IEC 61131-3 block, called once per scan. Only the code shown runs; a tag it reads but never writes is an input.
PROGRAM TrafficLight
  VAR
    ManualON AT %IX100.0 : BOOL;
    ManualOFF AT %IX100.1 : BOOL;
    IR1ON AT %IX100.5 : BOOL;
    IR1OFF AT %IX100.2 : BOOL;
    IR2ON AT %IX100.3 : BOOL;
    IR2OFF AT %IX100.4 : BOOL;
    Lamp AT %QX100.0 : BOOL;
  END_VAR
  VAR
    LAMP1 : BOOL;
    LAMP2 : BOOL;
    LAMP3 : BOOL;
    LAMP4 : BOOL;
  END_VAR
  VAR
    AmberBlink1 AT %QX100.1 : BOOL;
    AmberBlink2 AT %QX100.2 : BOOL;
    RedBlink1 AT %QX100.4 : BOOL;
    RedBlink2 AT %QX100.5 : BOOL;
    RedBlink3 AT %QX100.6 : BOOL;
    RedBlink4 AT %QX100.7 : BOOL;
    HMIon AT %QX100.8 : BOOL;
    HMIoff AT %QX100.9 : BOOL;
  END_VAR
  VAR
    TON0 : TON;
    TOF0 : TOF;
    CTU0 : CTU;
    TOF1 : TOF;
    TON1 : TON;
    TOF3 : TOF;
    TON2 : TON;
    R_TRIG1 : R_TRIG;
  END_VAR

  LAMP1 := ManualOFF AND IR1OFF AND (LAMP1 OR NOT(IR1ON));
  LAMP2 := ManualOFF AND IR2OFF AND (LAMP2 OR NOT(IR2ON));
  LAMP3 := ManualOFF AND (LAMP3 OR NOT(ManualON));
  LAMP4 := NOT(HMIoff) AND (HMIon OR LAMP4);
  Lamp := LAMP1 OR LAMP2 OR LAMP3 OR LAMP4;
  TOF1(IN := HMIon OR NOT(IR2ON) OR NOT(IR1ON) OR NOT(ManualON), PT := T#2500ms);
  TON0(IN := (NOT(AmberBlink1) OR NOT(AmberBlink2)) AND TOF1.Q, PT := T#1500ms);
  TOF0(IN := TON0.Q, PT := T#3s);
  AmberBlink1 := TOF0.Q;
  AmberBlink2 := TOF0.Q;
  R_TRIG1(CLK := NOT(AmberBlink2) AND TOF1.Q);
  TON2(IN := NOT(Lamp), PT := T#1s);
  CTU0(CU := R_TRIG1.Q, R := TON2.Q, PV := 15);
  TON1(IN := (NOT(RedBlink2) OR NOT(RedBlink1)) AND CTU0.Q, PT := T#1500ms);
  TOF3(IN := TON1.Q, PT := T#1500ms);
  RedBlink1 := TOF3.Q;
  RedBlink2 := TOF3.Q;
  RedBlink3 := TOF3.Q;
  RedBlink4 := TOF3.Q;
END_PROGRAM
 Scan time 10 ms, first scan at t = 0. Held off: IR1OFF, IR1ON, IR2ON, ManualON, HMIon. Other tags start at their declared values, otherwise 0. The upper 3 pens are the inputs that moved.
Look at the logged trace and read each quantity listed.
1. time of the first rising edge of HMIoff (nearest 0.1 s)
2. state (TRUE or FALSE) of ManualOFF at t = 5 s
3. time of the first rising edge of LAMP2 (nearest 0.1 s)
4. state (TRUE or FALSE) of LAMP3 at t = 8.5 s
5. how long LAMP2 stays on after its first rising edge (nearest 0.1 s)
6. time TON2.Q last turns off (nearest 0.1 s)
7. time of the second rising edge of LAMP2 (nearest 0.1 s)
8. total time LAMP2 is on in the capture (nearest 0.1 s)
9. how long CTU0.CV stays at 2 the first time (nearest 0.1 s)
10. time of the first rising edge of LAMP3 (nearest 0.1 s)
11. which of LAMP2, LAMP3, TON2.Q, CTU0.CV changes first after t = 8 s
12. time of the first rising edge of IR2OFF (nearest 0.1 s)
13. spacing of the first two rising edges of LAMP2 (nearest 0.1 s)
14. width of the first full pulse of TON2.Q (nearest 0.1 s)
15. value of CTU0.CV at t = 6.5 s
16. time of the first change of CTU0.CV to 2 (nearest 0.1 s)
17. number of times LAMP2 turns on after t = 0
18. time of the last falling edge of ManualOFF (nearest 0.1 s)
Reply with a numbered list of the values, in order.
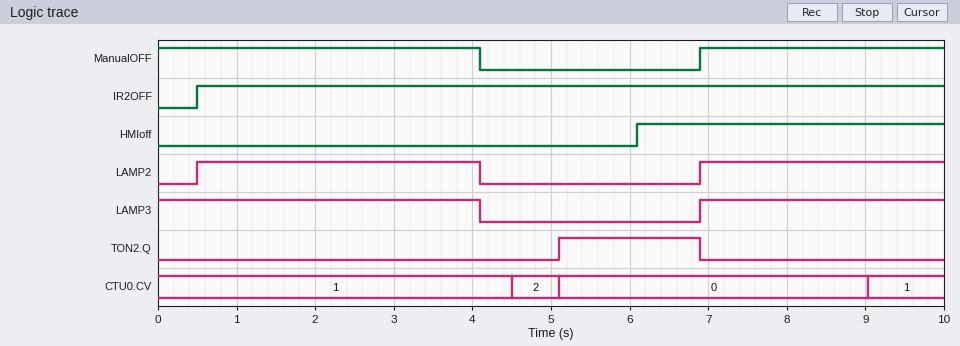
1. 6.1 s
2. FALSE
3. 0.5 s
4. TRUE
5. 3.6 s
6. 6.9 s
7. 6.9 s
8. 6.7 s
9. 0.6 s
10. 6.9 s
11. CTU0.CV
12. 0.5 s
13. 6.4 s
14. 1.8 s
15. 0
16. 4.5 s
17. 2
18. 4.1 s
